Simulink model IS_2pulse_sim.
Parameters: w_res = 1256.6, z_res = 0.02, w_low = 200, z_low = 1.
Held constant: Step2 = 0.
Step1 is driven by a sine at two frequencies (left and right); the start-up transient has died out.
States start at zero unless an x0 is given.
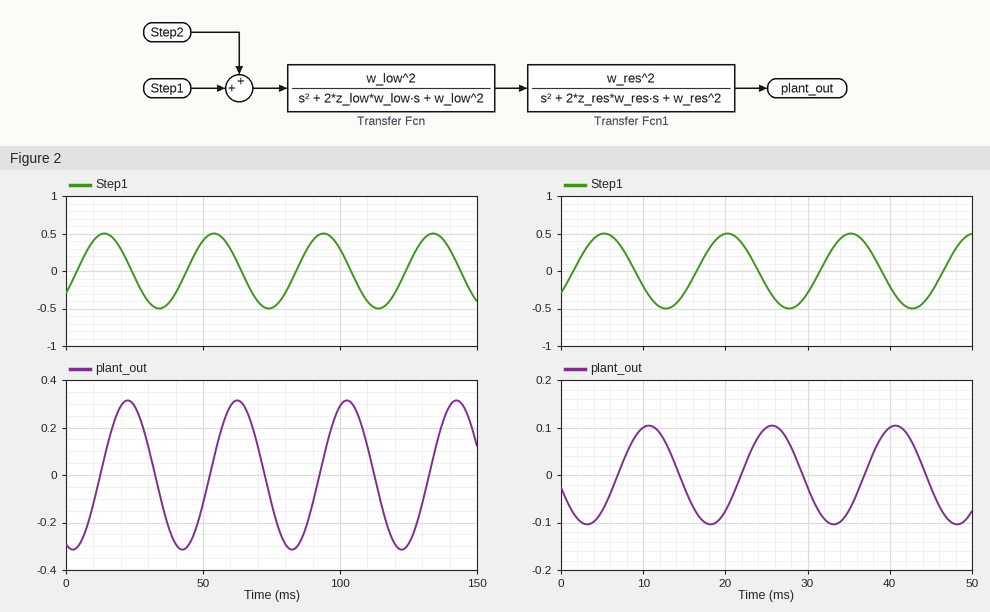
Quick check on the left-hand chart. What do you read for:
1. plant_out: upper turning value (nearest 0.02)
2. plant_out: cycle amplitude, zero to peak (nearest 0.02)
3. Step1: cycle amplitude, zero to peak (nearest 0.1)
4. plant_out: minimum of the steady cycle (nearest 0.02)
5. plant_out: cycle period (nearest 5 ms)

0.32
0.32
0.5
-0.32
40 ms
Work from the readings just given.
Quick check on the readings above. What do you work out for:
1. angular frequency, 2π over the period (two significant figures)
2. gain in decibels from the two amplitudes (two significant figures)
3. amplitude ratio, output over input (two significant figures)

0.16 rad/ms
-3.9 dB
0.64
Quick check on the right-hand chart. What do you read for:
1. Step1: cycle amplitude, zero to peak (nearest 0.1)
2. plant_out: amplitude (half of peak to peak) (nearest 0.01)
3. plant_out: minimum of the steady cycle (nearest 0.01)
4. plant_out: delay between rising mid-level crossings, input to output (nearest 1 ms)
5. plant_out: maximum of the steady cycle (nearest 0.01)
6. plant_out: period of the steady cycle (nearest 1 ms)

0.5
0.10
-0.10
5 ms
0.10
15 ms
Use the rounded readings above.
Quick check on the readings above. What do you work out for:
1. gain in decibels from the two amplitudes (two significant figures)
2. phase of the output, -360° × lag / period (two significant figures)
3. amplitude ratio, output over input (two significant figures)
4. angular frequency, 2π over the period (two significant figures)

-14 dB
-120°
0.20
0.42 rad/ms
